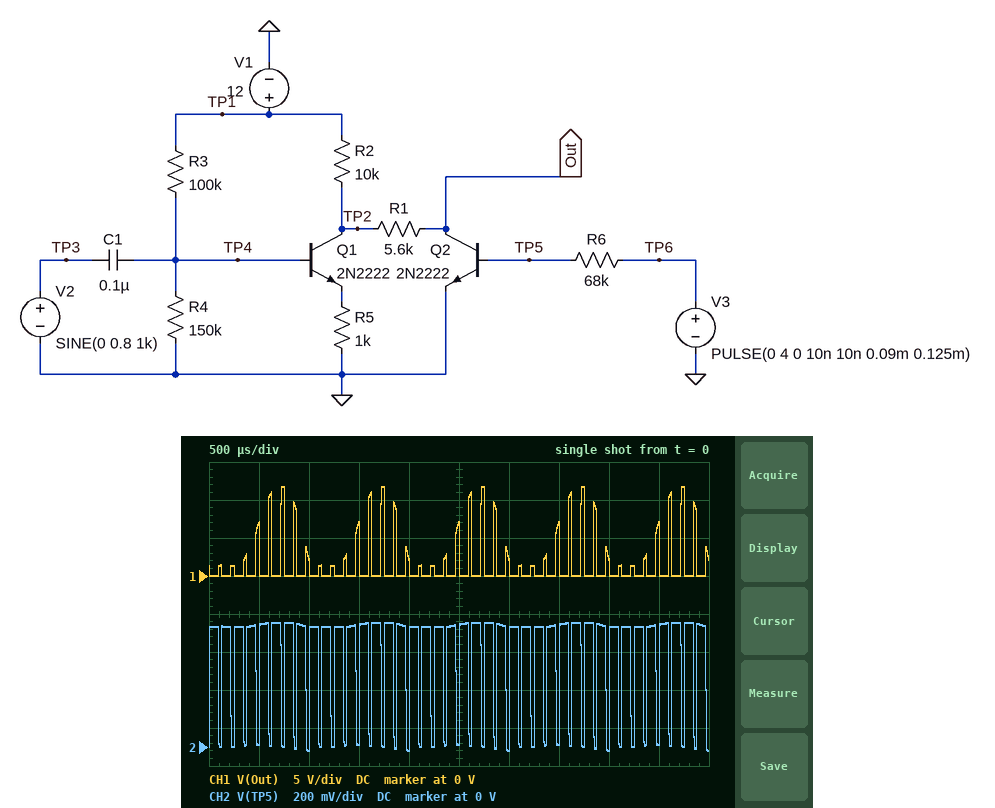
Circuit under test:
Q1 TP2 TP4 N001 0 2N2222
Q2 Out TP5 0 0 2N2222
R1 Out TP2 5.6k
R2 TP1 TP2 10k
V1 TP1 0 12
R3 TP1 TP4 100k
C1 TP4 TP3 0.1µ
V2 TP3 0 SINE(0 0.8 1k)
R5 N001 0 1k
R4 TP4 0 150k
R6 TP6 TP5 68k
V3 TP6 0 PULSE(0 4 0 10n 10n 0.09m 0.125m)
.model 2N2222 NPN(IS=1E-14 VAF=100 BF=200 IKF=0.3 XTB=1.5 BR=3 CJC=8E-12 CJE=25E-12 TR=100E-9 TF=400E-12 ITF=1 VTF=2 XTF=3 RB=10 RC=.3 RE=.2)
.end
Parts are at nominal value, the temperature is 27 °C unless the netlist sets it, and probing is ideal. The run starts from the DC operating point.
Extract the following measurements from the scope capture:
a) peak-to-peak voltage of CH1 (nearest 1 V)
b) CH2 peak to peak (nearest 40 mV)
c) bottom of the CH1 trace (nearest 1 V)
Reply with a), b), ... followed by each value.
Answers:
a) 12 V
b) 680 mV
c) 0 V
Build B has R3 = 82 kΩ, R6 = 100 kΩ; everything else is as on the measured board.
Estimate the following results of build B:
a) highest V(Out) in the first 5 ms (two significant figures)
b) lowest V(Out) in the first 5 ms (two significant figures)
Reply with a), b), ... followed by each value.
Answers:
a) 11 V
b) 27 mV
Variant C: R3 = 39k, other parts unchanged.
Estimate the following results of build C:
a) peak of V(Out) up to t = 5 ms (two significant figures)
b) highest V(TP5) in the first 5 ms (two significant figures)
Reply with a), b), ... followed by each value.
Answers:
a) 6.4 V
b) 640 mV
